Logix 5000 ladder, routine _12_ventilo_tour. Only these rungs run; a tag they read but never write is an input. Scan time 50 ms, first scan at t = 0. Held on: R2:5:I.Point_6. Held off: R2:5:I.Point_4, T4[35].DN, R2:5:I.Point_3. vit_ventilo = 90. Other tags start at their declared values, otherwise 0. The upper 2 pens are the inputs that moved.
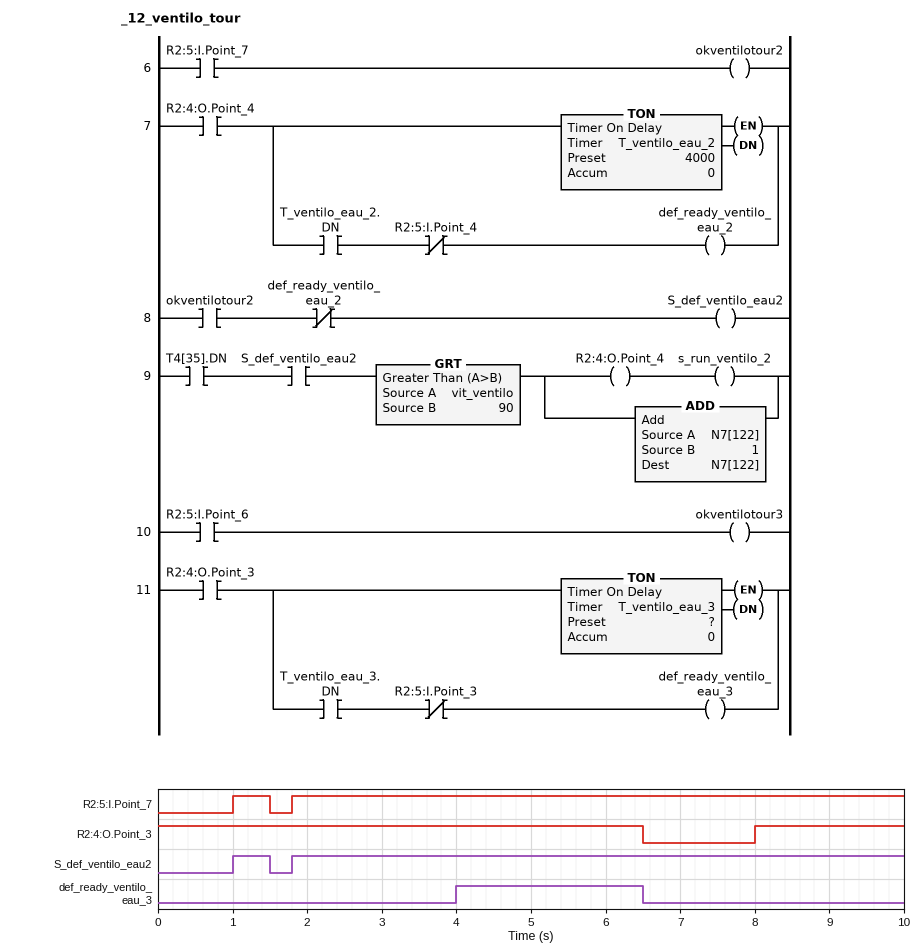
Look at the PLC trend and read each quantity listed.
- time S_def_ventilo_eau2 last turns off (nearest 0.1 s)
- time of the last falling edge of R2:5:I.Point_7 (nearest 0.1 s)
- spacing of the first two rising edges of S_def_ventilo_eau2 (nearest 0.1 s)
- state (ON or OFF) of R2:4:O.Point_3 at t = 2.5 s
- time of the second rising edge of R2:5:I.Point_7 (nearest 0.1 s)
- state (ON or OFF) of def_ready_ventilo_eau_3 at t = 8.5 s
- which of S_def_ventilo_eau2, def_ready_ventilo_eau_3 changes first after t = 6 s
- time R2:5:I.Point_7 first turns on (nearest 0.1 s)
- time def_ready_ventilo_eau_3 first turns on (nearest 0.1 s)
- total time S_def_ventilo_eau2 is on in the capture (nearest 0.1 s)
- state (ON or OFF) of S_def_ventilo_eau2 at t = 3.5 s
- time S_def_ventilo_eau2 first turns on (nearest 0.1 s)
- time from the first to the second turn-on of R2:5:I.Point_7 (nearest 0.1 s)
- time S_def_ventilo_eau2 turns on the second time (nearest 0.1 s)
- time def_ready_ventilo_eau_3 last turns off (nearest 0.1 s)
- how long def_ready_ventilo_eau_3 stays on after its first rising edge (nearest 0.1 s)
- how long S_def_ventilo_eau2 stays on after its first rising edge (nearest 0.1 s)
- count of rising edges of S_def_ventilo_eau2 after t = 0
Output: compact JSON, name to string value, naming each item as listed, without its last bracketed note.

{"time S_def_ventilo_eau2 last turns off": "1.5 s", "time of the last falling edge of R2:5:I.Point_7": "1.5 s", "spacing of the first two rising edges of S_def_ventilo_eau2": "0.8 s", "state (ON or OFF) of R2:4:O.Point_3 at t = 2.5 s": "ON", "time of the second rising edge of R2:5:I.Point_7": "1.8 s", "state (ON or OFF) of def_ready_ventilo_eau_3 at t = 8.5 s": "OFF", "which of S_def_ventilo_eau2, def_ready_ventilo_eau_3 changes first after t = 6 s": "def_ready_ventilo_eau_3", "time R2:5:I.Point_7 first turns on": "1.0 s", "time def_ready_ventilo_eau_3 first turns on": "4.0 s", "total time S_def_ventilo_eau2 is on in the capture": "8.7 s", "state (ON or OFF) of S_def_ventilo_eau2 at t = 3.5 s": "ON", "time S_def_ventilo_eau2 first turns on": "1.0 s", "time from the first to the second turn-on of R2:5:I.Point_7": "0.8 s", "time S_def_ventilo_eau2 turns on the second time": "1.8 s", "time def_ready_ventilo_eau_3 last turns off": "6.5 s", "how long def_ready_ventilo_eau_3 stays on after its first rising edge": "2.5 s", "how long S_def_ventilo_eau2 stays on after its first rising edge": "0.5 s", "count of rising edges of S_def_ventilo_eau2 after t = 0": "2"}
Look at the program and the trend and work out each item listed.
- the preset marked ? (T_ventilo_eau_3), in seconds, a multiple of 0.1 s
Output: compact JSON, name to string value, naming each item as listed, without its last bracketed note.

{"the preset marked ? (T_ventilo_eau_3), in seconds, a multiple of 0.1 s": "4.0 s"}
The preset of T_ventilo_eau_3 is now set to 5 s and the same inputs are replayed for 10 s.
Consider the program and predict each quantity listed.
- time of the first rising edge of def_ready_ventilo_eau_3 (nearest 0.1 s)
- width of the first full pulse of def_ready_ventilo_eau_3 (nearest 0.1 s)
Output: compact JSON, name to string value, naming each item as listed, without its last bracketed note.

{"time of the first rising edge of def_ready_ventilo_eau_3": "5.0 s", "width of the first full pulse of def_ready_ventilo_eau_3": "1.5 s"}
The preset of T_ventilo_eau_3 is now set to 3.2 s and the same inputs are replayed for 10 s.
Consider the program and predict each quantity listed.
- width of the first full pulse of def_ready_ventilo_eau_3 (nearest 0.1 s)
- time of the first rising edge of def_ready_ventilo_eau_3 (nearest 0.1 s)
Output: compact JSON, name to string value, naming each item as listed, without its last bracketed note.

{"width of the first full pulse of def_ready_ventilo_eau_3": "3.3 s", "time of the first rising edge of def_ready_ventilo_eau_3": "3.2 s"}
